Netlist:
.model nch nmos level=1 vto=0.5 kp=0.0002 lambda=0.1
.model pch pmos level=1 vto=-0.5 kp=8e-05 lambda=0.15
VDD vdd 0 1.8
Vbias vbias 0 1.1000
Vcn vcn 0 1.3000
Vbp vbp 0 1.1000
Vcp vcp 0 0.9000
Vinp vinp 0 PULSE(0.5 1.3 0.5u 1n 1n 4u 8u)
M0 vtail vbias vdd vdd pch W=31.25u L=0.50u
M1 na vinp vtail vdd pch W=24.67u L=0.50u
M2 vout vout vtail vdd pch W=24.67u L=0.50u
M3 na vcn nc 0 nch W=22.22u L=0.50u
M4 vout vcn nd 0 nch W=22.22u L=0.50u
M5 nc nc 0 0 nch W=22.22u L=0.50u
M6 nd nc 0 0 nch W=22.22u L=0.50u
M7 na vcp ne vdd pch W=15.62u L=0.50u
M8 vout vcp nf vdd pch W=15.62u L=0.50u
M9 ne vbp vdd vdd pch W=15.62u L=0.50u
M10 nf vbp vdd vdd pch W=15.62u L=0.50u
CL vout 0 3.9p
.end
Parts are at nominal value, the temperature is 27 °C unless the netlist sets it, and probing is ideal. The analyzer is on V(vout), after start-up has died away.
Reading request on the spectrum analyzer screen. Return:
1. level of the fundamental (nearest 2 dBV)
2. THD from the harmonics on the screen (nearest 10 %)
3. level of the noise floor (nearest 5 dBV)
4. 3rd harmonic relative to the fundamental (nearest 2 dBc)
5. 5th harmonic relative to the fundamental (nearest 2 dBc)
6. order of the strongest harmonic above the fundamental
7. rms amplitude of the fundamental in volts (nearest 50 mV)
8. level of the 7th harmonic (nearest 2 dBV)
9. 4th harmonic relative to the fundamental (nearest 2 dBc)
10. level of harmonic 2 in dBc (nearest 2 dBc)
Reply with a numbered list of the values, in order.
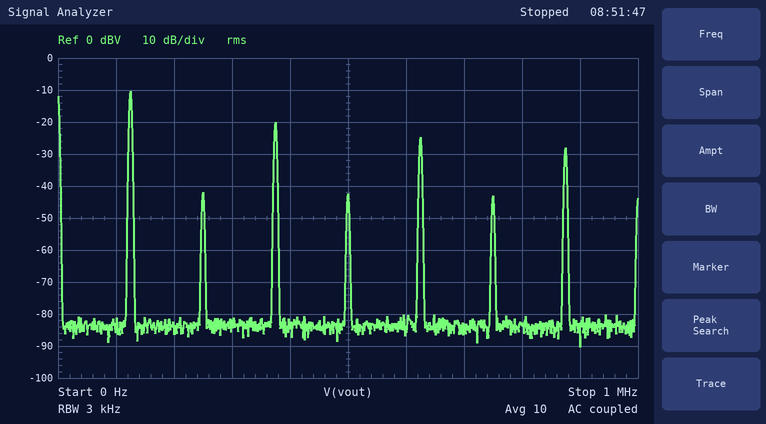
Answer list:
1. -10 dBV
2. 40 %
3. -85 dBV
4. -10 dBc
5. -14 dBc
6. 3
7. 300 mV
8. -28 dBV
9. -32 dBc
10. -32 dBc
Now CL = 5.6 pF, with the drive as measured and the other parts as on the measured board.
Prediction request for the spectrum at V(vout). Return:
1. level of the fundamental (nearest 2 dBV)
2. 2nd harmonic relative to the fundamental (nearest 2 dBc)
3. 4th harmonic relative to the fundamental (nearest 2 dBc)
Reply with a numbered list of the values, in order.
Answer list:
1. -10 dBV
2. -28 dBc
3. -30 dBc
